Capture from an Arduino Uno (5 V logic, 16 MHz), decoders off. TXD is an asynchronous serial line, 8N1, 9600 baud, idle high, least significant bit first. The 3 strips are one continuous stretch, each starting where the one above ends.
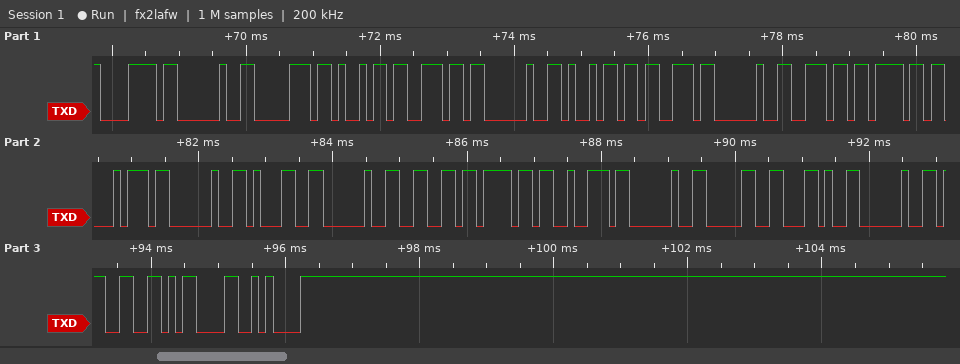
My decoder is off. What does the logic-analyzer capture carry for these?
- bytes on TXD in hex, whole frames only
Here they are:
0x78 0x20 0x70 0x69 0x6E 0x20 0x69 0x73 0x20 0x6E 0x6F 0x74 0x20 0x31 0x20 0x66 0x6F 0x72 0x20 0x30 0x2C 0x20 0x33 0x0D 0x0A
